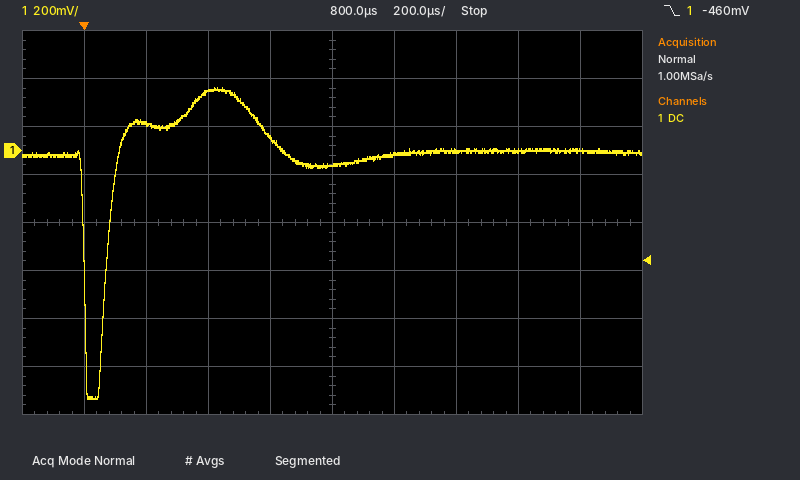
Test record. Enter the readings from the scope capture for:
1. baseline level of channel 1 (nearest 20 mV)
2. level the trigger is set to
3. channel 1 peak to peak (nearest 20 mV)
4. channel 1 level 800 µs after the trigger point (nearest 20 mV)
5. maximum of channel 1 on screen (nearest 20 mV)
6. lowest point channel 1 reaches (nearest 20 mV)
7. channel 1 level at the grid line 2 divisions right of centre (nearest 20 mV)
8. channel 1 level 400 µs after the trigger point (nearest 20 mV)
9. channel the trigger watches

0 mV
-460 mV
1.30 V
-60 mV
260 mV
-1.04 V
0 mV
240 mV
channel 1
